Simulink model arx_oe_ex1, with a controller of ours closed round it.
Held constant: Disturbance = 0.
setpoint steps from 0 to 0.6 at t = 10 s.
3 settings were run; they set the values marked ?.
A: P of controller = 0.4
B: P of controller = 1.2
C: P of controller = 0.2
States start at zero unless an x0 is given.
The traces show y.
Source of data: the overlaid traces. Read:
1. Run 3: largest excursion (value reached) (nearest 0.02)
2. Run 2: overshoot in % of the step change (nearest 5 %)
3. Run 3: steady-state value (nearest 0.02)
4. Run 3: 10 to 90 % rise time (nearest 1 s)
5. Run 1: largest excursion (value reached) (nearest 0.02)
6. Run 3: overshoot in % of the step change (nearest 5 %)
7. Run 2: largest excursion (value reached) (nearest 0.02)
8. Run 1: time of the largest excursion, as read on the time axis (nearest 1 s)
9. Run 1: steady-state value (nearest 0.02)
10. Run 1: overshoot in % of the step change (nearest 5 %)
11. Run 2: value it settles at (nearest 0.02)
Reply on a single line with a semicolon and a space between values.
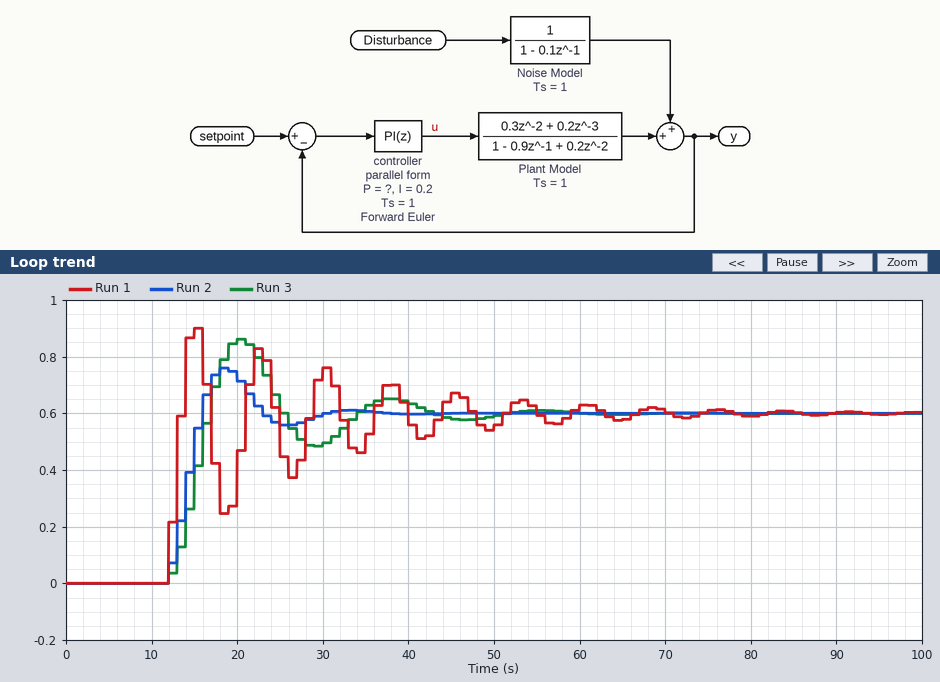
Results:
0.86; 25 %; 0.60; 3 s; 0.90; 45 %; 0.76; 15 s; 0.60; 50 %; 0.60
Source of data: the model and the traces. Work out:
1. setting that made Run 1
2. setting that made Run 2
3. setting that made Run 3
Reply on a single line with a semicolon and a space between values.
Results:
B; A; C
